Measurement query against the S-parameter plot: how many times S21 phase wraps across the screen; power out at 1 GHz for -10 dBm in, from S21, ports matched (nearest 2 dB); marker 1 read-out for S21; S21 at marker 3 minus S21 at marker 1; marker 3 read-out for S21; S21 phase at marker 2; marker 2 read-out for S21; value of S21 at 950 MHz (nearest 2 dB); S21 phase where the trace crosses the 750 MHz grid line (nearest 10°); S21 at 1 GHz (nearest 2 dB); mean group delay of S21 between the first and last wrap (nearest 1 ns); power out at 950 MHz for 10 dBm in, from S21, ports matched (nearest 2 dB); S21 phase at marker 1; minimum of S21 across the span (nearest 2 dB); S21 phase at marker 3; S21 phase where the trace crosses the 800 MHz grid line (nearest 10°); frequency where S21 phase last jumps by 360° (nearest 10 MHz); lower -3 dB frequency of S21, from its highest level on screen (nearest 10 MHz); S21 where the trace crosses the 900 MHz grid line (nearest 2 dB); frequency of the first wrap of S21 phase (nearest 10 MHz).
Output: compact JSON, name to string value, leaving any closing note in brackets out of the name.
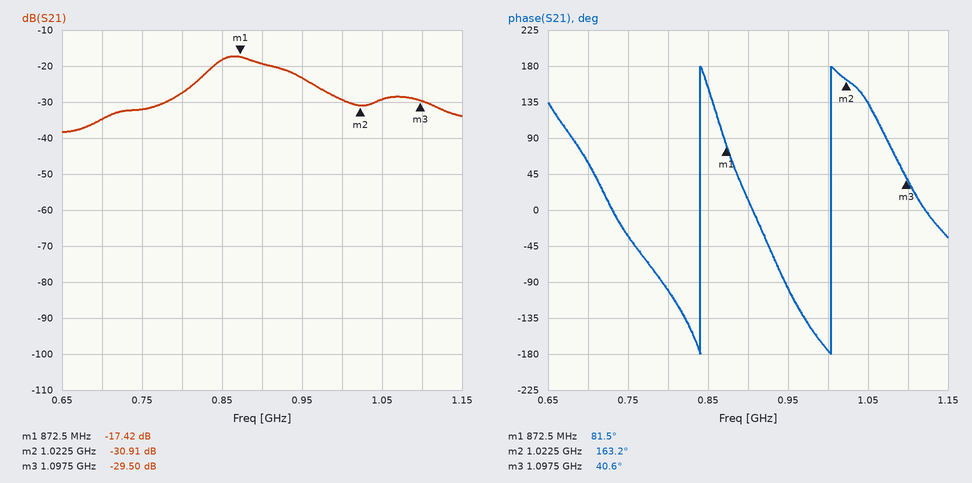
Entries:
{"how many times S21 phase wraps across the screen": "2", "power out at 1 GHz for -10 dBm in, from S21, ports matched": "-40 dBm", "marker 1 read-out for S21": "-17.42 dB", "S21 at marker 3 minus S21 at marker 1": "-12.08 dB", "marker 3 read-out for S21": "-29.50 dB", "S21 phase at marker 2": "163.2°", "marker 2 read-out for S21": "-30.91 dB", "value of S21 at 950 MHz": "-24 dB", "S21 phase where the trace crosses the 750 MHz grid line": "-30°", "S21 at 1 GHz": "-30 dB", "mean group delay of S21 between the first and last wrap": "6 ns", "power out at 950 MHz for 10 dBm in, from S21, ports matched": "-14 dBm", "S21 phase at marker 1": "81.5°", "minimum of S21 across the span": "-38 dB", "S21 phase at marker 3": "40.6°", "S21 phase where the trace crosses the 800 MHz grid line": "-100°", "frequency where S21 phase last jumps by 360°": "1.00 GHz", "lower -3 dB frequency of S21, from its highest level on screen": "840 MHz", "S21 where the trace crosses the 900 MHz grid line": "-20 dB", "frequency of the first wrap of S21 phase": "840 MHz"}
